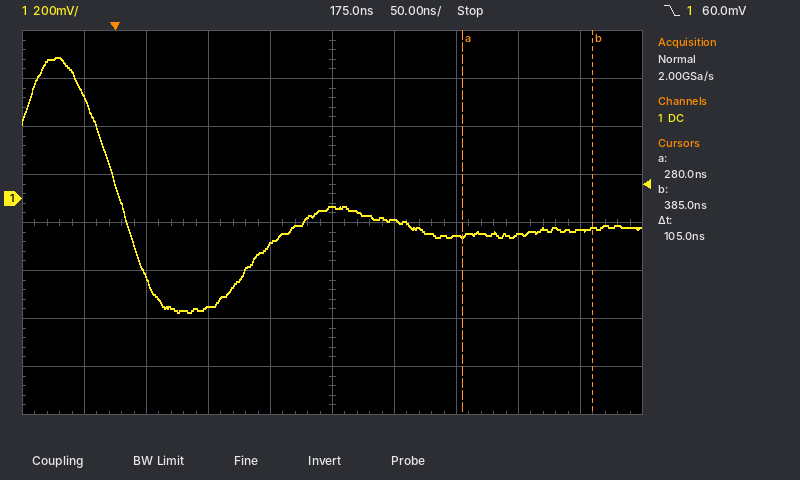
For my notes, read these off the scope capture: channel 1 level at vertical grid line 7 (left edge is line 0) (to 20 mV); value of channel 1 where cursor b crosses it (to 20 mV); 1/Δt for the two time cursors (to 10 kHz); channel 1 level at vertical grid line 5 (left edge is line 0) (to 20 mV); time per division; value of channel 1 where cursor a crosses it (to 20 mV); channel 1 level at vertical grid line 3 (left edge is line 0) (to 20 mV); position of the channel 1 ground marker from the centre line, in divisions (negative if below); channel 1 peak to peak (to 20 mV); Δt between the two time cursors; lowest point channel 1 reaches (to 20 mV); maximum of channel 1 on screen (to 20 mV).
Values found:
-160 mV
-120 mV
9.52 MHz
-40 mV
50 ns
-160 mV
-460 mV
+0.5 div
1.06 V
105 ns
-480 mV
580 mV
